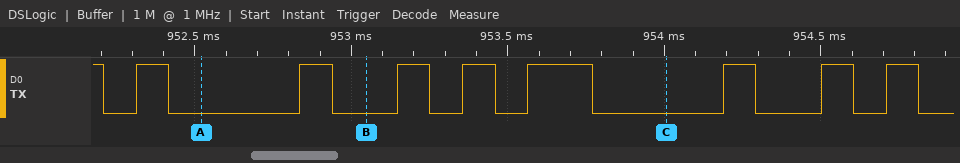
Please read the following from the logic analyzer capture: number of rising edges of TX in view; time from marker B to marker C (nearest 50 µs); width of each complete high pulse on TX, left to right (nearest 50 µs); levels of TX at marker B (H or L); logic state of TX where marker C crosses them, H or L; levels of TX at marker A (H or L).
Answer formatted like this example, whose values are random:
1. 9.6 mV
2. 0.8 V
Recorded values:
1. 8
2. 950 µs
3. 100 µs, 100 µs, 100 µs, 100 µs, 200 µs, 100 µs, 100 µs, 100 µs
4. TX=L
5. TX=L
6. TX=L
